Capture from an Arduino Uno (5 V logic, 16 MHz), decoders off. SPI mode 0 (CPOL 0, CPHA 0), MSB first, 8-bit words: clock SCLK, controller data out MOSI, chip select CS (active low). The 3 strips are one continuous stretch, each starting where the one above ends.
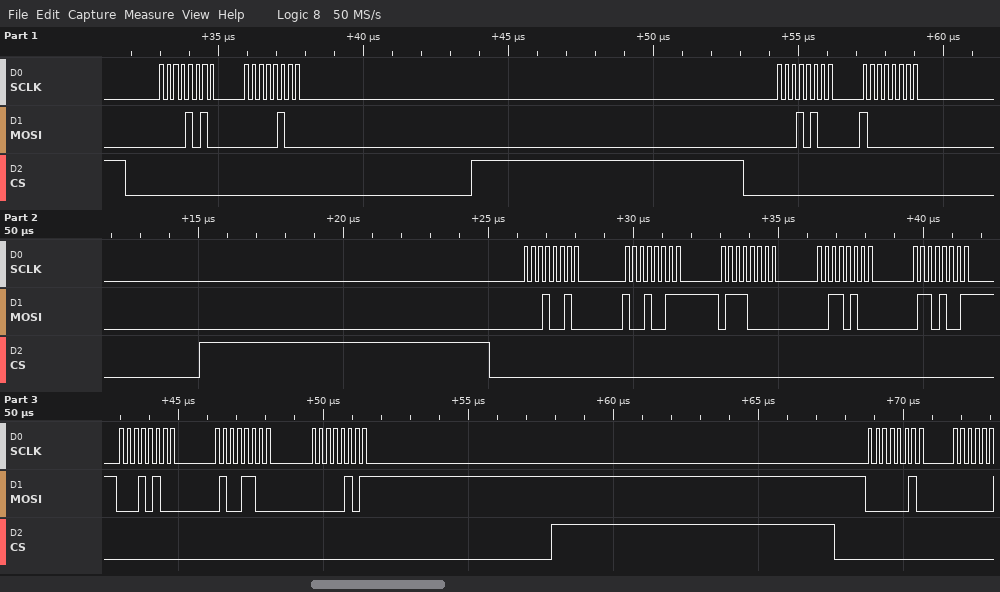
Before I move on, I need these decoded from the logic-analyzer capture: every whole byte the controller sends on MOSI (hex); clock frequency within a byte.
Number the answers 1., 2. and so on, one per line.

1. 0x0A 0x04 0x14 0x80 0x12 0x93 0x70 0x34 0x69 0x14 0x4C 0x05 0x02
2. 4 MHz
